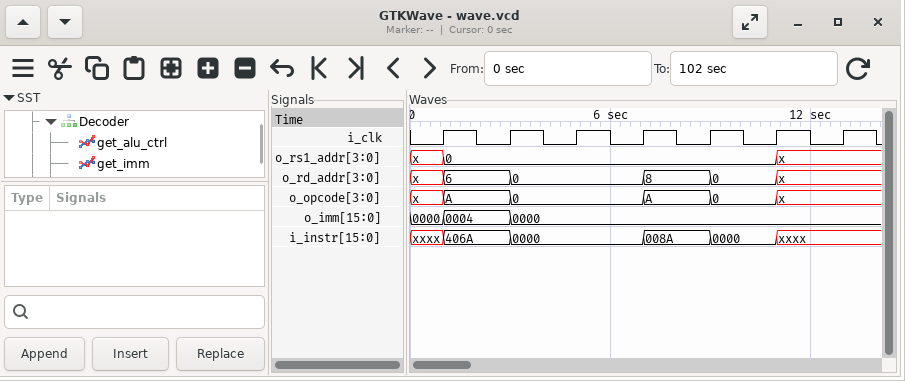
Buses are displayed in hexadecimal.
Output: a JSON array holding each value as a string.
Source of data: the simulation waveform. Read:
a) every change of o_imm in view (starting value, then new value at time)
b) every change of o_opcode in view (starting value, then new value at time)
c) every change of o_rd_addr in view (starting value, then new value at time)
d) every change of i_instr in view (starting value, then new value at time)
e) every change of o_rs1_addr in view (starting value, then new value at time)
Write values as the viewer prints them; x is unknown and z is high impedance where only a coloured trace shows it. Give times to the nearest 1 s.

["0000, 0004 at 1 s, 0000 at 3 s", "x, A at 1 s, 0 at 3 s, A at 7 s, 0 at 9 s, x at 11 s", "x, 6 at 1 s, 0 at 3 s, 8 at 7 s, 0 at 9 s, x at 11 s", "xxxx, 406A at 1 s, 0000 at 3 s, 008A at 7 s, 0000 at 9 s, xxxx at 11 s", "x, 0 at 1 s, x at 11 s"]
